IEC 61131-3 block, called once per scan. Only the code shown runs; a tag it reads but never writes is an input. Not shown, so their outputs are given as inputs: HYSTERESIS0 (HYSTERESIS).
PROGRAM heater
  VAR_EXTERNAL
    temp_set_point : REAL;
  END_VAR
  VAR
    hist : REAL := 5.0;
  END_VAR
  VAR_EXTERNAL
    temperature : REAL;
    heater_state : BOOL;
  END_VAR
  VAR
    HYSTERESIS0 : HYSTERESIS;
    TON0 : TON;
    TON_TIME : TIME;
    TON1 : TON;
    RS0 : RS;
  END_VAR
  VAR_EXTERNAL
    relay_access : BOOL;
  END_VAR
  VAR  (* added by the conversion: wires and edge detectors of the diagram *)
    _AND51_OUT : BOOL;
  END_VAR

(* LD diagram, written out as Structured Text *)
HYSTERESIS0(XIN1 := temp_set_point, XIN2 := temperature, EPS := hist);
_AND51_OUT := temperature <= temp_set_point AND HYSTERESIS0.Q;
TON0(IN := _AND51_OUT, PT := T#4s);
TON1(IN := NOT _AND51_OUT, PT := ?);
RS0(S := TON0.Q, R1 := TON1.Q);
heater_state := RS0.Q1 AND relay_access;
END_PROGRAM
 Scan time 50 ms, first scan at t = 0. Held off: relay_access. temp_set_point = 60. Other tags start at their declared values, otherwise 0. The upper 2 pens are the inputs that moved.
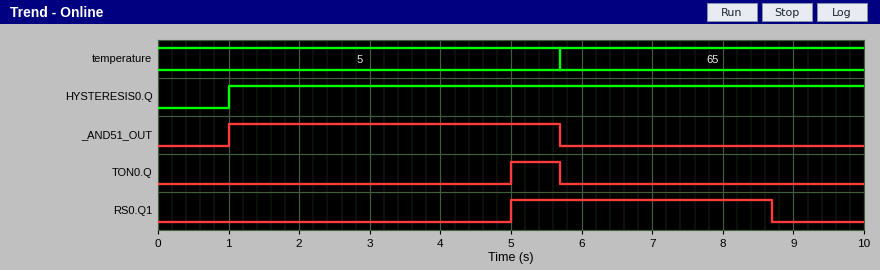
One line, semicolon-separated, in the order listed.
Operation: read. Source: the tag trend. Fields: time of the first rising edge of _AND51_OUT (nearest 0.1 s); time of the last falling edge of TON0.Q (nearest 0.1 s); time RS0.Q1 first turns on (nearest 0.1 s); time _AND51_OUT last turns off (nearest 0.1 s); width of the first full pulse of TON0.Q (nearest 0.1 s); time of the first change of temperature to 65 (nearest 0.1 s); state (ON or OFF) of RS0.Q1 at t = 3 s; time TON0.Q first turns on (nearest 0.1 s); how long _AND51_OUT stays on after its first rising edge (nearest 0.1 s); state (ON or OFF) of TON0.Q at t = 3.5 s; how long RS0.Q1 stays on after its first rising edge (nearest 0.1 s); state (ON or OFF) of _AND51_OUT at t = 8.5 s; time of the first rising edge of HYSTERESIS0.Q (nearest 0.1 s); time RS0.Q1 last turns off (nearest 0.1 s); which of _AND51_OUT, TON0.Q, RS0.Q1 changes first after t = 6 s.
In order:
1.0 s; 5.7 s; 5.0 s; 5.7 s; 0.7 s; 5.7 s; OFF; 5.0 s; 4.7 s; OFF; 3.7 s; OFF; 1.0 s; 8.7 s; RS0.Q1
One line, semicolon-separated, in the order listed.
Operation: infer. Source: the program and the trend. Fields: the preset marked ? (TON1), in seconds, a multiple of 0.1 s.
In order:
3.0 s
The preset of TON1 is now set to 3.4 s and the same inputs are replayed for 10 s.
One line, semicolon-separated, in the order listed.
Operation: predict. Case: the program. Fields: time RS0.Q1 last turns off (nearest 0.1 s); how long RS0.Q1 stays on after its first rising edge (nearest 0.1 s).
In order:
9.1 s; 4.1 s
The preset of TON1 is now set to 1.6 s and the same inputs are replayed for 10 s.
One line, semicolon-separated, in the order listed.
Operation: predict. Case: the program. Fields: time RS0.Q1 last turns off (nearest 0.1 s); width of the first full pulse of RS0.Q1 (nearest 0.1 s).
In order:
7.3 s; 2.3 s
